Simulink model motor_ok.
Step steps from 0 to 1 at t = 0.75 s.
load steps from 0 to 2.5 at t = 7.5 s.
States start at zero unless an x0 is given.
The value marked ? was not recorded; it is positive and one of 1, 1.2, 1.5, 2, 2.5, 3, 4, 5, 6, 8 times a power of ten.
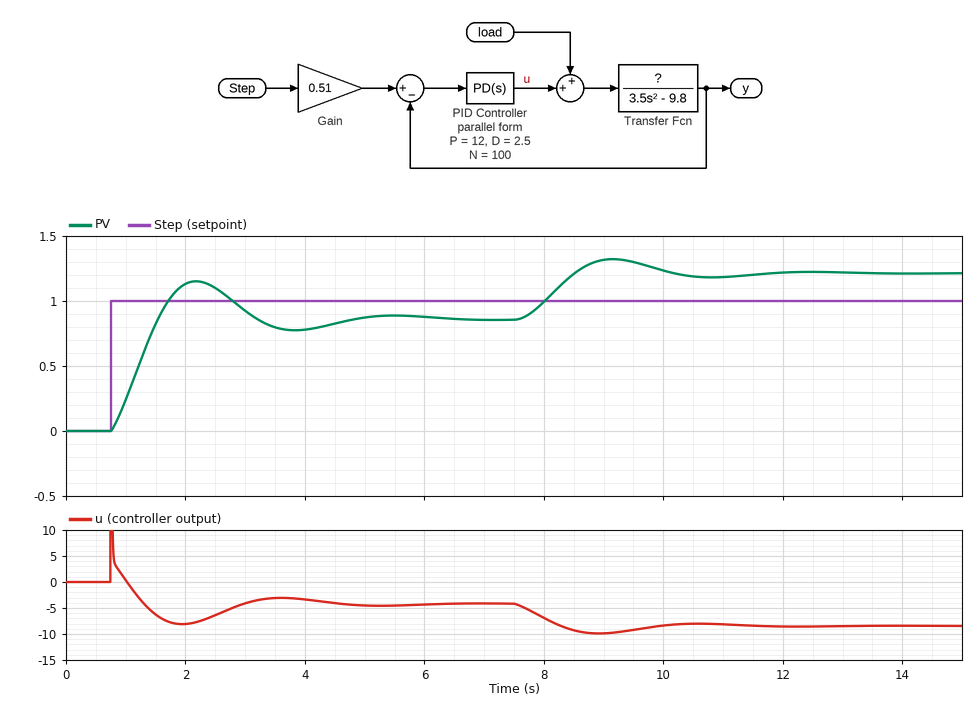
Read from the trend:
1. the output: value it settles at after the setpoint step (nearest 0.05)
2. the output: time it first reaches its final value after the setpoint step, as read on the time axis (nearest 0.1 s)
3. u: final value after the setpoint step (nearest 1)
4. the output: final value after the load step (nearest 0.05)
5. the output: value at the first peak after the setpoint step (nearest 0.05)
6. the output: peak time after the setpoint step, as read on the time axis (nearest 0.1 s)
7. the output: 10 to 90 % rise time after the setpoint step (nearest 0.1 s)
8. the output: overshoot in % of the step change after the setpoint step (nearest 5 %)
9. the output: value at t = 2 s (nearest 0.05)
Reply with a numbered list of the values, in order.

1. 0.85
2. 1.5 s
3. -4
4. 1.20
5. 1.15
6. 2.2 s
7. 0.6 s
8. 35 %
9. 1.15
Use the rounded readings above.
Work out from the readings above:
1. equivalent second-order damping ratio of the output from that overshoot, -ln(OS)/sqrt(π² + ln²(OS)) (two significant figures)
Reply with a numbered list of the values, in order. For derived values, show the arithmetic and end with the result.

1. ln(0.35) = -1.050; 1.050 / sqrt(9.870 + 1.102) = 0.32
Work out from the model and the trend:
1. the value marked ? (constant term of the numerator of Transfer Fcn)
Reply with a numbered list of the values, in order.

1. 2
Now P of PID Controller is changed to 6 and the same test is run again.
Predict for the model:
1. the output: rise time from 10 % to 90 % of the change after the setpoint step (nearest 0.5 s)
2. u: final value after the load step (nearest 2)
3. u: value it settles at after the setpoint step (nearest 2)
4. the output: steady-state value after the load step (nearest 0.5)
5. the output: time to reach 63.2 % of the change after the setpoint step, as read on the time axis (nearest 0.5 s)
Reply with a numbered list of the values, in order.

1. 3.5 s
2. -28
3. -14
4. 5.0
5. 3.0 s
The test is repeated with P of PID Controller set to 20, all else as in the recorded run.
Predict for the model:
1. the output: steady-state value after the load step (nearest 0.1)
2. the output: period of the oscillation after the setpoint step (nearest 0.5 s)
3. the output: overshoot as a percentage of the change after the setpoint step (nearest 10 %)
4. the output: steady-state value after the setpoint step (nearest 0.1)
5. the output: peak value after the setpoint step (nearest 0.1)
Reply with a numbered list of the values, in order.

1. 0.8
2. 2.0 s
3. 50 %
4. 0.7
5. 1.0
